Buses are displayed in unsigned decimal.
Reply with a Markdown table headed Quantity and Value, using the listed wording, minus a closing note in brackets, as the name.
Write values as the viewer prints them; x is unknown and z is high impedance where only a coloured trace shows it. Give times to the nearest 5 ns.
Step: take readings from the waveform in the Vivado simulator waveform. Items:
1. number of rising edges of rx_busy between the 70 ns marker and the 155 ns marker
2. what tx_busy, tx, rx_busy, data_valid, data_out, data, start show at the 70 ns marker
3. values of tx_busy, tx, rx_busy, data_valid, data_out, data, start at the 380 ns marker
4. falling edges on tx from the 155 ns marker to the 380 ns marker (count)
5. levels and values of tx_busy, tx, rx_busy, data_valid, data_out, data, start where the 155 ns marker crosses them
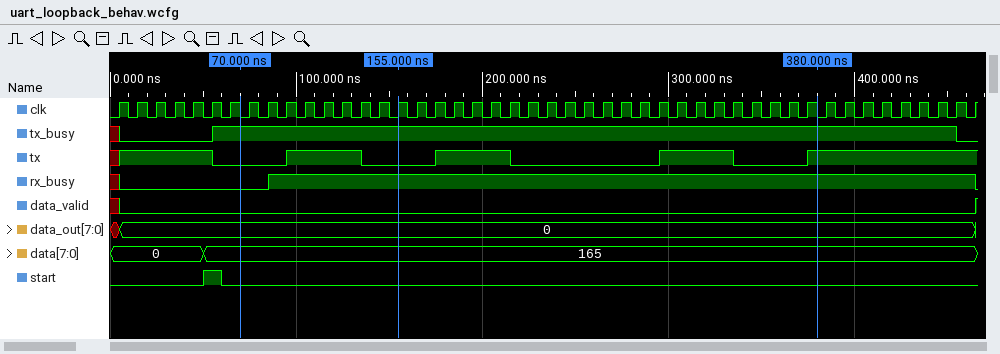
| Quantity | Value |
|---|---|
| number of rising edges of rx_busy between the 70 ns marker and the 155 ns marker | 1 |
| what tx_busy, tx, rx_busy, data_valid, data_out, data, start show at the 70 ns marker | tx_busy=1, tx=0, rx_busy=0, data_valid=0, data_out=0, data=165, start=0 |
| values of tx_busy, tx, rx_busy, data_valid, data_out, data, start at the 380 ns marker | tx_busy=1, tx=1, rx_busy=1, data_valid=0, data_out=0, data=165, start=0 |
| falling edges on tx from the 155 ns marker to the 380 ns marker | 2 |
| levels and values of tx_busy, tx, rx_busy, data_valid, data_out, data, start where the 155 ns marker crosses them | tx_busy=1, tx=0, rx_busy=1, data_valid=0, data_out=0, data=165, start=0 |
